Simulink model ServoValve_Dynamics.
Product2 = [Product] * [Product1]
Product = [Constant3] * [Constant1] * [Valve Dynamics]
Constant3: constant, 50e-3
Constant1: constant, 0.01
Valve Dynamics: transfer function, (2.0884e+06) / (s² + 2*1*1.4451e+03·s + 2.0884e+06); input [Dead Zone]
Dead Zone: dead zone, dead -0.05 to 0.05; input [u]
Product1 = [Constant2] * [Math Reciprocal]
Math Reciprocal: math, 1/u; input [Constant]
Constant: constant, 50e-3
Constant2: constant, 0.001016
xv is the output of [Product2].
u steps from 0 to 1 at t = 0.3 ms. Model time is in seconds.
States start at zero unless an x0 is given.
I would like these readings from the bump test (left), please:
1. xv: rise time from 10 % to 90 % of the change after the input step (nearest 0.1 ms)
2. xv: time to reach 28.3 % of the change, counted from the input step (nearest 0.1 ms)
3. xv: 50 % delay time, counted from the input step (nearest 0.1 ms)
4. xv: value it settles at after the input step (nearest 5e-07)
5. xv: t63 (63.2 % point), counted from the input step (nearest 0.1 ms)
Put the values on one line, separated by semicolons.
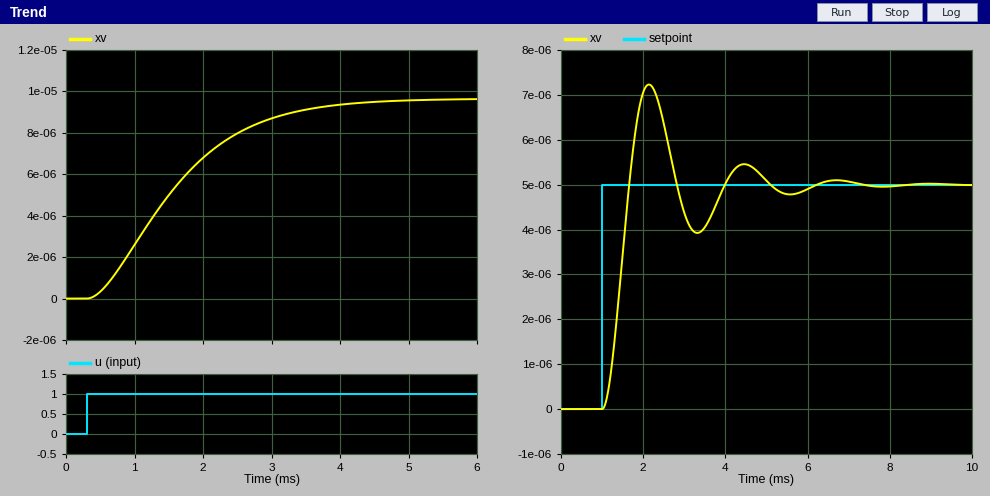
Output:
2.3 ms; 0.7 ms; 1.2 ms; 0.0000095; 1.5 ms
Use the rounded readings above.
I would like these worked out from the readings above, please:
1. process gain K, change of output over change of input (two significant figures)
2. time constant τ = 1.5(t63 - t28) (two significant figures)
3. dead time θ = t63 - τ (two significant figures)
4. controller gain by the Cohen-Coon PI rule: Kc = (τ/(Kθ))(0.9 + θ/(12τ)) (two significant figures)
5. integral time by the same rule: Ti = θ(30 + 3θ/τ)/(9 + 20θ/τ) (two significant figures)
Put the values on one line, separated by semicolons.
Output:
0.0000095; 1.2 ms; 0.30 ms; 390000; 0.66 ms
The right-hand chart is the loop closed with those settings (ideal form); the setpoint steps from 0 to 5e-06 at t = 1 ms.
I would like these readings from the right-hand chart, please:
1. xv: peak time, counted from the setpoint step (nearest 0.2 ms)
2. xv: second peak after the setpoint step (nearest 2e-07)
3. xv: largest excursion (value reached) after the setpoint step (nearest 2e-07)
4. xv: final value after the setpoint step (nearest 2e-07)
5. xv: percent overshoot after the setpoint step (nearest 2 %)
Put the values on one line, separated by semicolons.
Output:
1.2 ms; 0.0000054; 0.0000072; 0.0000050; 44 %
